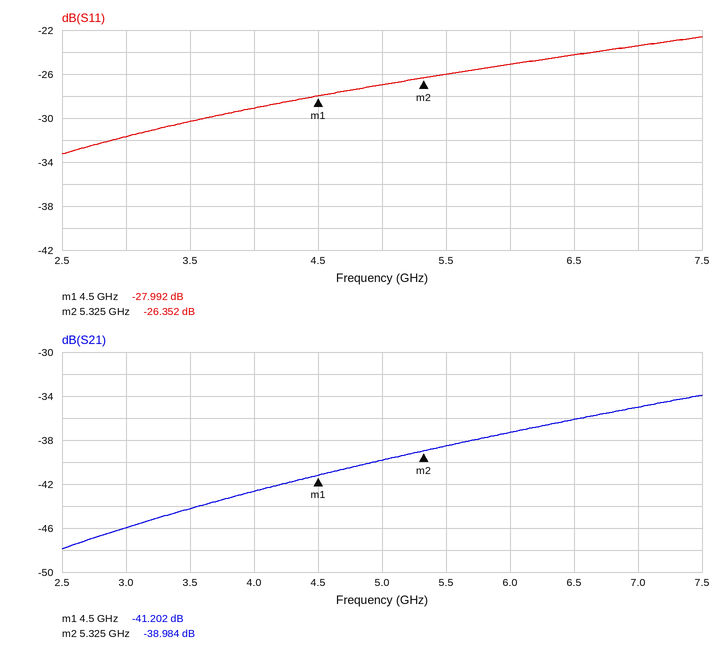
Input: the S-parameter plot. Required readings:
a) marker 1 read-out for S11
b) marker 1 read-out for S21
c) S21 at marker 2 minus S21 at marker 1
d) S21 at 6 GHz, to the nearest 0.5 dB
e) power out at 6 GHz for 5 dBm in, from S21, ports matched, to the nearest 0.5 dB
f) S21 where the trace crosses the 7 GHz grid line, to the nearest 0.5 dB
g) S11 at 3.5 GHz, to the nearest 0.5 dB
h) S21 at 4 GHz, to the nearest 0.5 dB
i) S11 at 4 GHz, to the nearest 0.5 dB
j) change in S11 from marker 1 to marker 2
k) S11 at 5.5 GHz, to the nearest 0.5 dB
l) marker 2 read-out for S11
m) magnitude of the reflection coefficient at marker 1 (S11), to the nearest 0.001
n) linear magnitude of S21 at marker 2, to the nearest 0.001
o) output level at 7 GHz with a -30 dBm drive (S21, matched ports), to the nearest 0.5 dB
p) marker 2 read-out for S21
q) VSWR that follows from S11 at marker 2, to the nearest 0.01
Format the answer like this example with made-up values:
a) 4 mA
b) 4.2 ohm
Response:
a) -27.992 dB
b) -41.202 dB
c) 2.218 dB
d) -37.5 dB
e) -32.5 dBm
f) -35.0 dB
g) -30.5 dB
h) -42.5 dB
i) -29.0 dB
j) 1.640 dB
k) -26.0 dB
l) -26.352 dB
m) 0.040
n) 0.011
o) -65.0 dBm
p) -38.984 dB
q) 1.10
